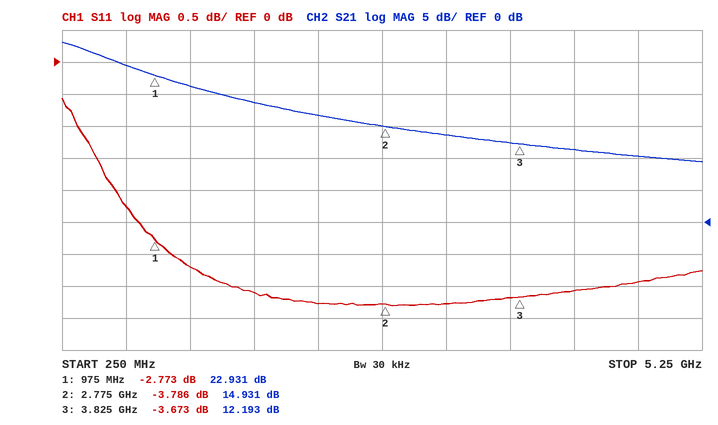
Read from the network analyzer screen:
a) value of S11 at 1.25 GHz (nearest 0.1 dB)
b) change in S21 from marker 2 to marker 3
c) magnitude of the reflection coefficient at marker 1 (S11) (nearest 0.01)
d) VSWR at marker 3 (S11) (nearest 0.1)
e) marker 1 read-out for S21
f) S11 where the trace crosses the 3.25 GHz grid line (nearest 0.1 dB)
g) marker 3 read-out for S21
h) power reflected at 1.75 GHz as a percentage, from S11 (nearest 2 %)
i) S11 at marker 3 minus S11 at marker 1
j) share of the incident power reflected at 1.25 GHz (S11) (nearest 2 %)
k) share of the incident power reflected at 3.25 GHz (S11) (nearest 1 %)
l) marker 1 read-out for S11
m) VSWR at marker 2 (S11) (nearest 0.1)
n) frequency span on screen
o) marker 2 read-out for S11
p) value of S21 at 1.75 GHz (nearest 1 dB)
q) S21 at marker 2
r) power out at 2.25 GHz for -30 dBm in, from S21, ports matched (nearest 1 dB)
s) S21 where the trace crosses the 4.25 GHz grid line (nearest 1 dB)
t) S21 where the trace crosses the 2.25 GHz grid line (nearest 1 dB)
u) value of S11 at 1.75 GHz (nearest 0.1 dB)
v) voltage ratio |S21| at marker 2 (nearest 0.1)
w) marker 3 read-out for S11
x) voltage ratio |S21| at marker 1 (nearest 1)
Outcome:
-3.2 dB
-2.738 dB
0.73
4.8
22.931 dB
-3.8 dB
12.193 dB
44 %
-0.900 dB
48 %
42 %
-2.773 dB
4.7
5 GHz
-3.786 dB
19 dB
14.931 dB
-13 dBm
11 dB
17 dB
-3.6 dB
5.6
-3.673 dB
14
